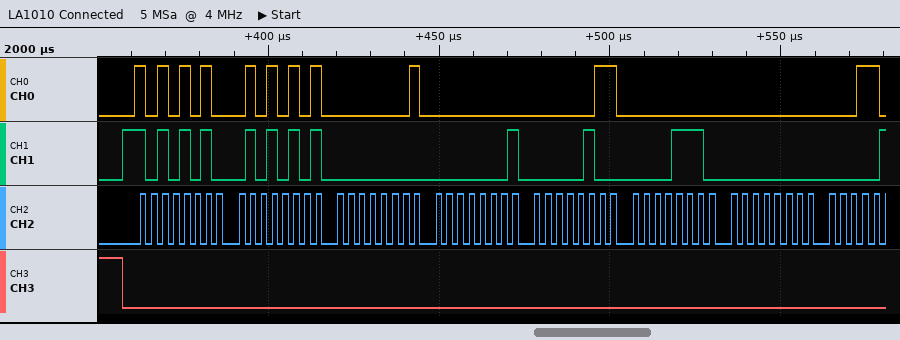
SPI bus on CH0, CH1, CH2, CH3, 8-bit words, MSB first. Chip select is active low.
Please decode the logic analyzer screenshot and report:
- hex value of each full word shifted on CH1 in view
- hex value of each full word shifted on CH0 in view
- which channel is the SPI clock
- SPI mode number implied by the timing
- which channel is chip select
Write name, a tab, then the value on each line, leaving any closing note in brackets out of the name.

hex value of each full word shifted on CH1 in view	AA, 55, 00, 01, 04, 0E, 00
hex value of each full word shifted on CH0 in view	AA, 55, 01, 00, 03, 00, 00
which channel is the SPI clock	CH2
SPI mode number implied by the timing	0
which channel is chip select	CH3
